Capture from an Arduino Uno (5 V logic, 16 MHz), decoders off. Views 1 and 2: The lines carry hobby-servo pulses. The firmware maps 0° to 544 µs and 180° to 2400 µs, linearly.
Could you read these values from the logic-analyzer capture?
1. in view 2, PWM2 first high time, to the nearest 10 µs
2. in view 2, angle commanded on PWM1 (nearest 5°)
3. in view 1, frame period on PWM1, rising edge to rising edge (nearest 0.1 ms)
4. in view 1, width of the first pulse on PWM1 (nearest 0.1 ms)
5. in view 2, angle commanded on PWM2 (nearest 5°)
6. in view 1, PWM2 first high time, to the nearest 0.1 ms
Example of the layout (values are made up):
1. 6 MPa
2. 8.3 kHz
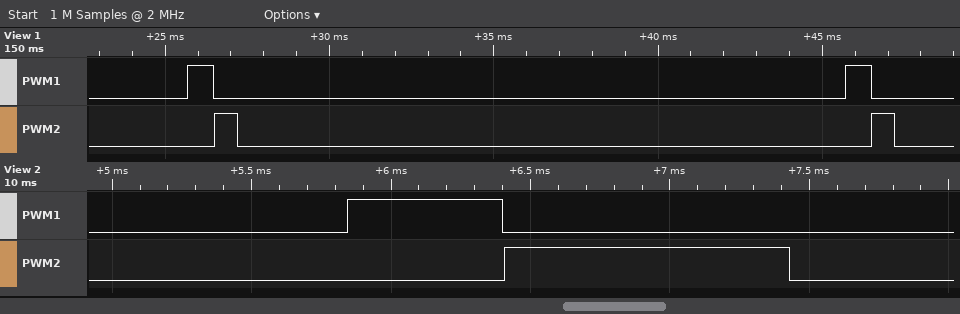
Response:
1. 1020 µs
2. 0°
3. 20.0 ms
4. 0.8 ms
5. 45°
6. 0.7 ms
